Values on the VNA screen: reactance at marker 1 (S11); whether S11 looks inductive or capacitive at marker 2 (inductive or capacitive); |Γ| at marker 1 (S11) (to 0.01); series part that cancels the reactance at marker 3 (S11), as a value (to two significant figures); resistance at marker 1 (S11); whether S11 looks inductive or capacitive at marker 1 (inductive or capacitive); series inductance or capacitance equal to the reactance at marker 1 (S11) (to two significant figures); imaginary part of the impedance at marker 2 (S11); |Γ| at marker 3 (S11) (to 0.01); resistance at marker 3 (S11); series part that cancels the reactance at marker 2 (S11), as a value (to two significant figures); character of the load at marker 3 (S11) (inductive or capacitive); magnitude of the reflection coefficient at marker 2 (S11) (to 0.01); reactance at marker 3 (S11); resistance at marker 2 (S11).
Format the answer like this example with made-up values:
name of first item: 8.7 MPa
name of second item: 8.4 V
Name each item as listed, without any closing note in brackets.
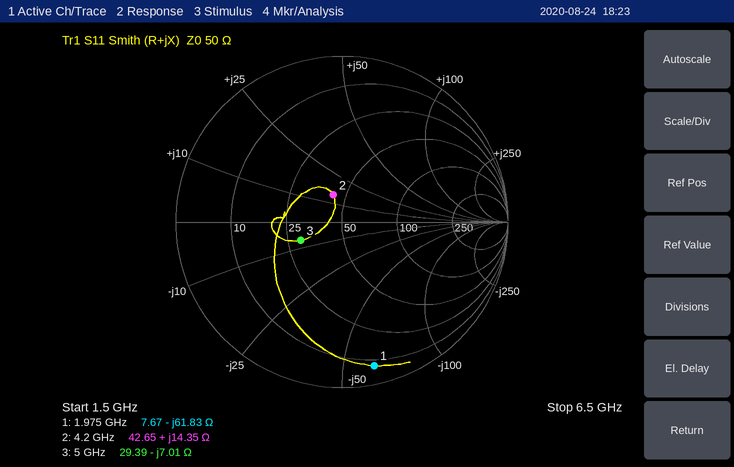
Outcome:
reactance at marker 1: -61.83 Ω
whether S11 looks inductive or capacitive at marker 2: inductive
|Γ| at marker 1 (S11): 0.89
series part that cancels the reactance at marker 3 (S11), as a value: 220 pH
resistance at marker 1: 7.67 Ω
whether S11 looks inductive or capacitive at marker 1: capacitive
series inductance or capacitance equal to the reactance at marker 1 (S11): 1.3 pF
imaginary part of the impedance at marker 2: +14.35 Ω
|Γ| at marker 3 (S11): 0.27
resistance at marker 3: 29.39 Ω
series part that cancels the reactance at marker 2 (S11), as a value: 2.6 pF
character of the load at marker 3 (S11): capacitive
magnitude of the reflection coefficient at marker 2 (S11): 0.17
reactance at marker 3: -7.01 Ω
resistance at marker 2: 42.65 Ω
